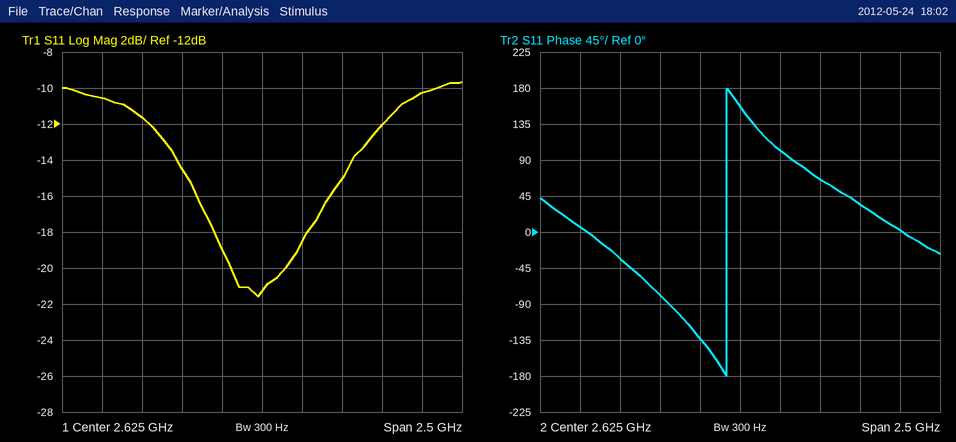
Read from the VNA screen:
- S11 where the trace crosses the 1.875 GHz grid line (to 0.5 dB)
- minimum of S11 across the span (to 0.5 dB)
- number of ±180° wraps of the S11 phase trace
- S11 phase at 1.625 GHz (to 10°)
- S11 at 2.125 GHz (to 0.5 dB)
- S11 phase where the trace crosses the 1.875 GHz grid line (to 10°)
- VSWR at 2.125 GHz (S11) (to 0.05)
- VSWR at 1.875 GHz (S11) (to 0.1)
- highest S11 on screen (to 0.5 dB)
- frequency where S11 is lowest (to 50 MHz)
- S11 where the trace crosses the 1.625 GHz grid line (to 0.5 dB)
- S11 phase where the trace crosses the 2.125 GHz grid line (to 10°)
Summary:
-11.5 dB
-21.5 dB
1
10°
-14.5 dB
-30°
1.45
1.7
-9.5 dB
2.60 GHz
-10.5 dB
-80°
